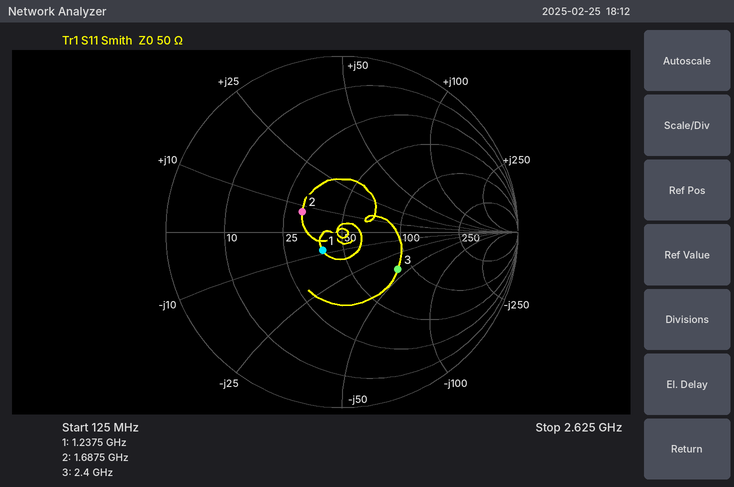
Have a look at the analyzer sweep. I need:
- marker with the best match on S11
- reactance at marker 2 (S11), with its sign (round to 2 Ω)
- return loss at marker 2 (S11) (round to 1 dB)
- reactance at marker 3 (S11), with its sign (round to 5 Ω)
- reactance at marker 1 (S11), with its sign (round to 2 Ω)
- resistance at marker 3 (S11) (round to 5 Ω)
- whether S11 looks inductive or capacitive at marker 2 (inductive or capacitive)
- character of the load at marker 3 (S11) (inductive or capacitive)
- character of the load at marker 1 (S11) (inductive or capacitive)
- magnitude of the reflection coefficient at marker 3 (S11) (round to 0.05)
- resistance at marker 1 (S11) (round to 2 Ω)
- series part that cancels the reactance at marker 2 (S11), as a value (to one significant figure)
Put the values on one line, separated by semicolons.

marker 1; +8 Ω; 12 dB; -40 Ω; -8 Ω; 85 Ω; inductive; capacitive; capacitive; 0.40; 40 Ω; 10 pF
